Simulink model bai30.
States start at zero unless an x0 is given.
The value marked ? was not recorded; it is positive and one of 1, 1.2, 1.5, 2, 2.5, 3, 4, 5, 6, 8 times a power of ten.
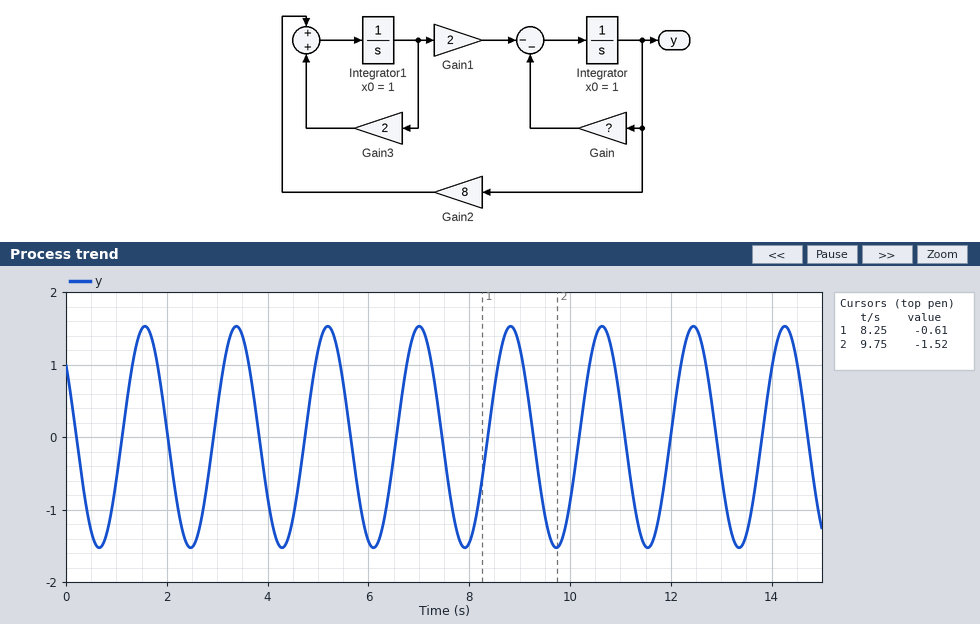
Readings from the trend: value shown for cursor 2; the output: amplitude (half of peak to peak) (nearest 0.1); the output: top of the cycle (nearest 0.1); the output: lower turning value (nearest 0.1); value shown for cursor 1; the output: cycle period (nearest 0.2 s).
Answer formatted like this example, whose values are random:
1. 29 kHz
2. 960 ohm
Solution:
1. -1.52
2. 1.5
3. 1.5
4. -1.5
5. -0.61
6. 1.8 s
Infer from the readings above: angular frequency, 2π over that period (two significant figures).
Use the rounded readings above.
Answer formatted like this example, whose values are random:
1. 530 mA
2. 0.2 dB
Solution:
1. 3.5 rad/s
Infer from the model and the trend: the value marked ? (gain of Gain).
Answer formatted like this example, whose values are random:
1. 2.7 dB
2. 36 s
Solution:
1. 2
